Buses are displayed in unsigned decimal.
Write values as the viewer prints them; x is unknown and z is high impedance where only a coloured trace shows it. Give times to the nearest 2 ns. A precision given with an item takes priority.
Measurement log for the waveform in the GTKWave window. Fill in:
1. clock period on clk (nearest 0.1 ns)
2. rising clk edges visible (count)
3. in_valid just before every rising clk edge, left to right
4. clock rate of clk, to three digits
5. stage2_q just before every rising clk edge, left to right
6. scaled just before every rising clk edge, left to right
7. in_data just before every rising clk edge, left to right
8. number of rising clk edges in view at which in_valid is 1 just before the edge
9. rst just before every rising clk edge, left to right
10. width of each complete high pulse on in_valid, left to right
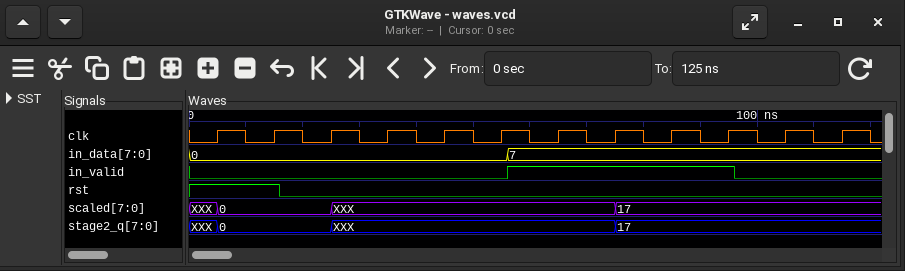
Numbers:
10 ns
12
0 0 0 0 0 0 1 1 1 1 0 0
100 MHz
XXX, 0, 0, XXX, XXX, XXX, XXX, XXX, 17, 17, 17, 17
XXX, 0, 0, XXX, XXX, XXX, XXX, XXX, 17, 17, 17, 17
0, 0, 0, 0, 0, 0, 7, 7, 7, 7, 7, 7
4
1 1 0 0 0 0 0 0 0 0 0 0
40 ns
